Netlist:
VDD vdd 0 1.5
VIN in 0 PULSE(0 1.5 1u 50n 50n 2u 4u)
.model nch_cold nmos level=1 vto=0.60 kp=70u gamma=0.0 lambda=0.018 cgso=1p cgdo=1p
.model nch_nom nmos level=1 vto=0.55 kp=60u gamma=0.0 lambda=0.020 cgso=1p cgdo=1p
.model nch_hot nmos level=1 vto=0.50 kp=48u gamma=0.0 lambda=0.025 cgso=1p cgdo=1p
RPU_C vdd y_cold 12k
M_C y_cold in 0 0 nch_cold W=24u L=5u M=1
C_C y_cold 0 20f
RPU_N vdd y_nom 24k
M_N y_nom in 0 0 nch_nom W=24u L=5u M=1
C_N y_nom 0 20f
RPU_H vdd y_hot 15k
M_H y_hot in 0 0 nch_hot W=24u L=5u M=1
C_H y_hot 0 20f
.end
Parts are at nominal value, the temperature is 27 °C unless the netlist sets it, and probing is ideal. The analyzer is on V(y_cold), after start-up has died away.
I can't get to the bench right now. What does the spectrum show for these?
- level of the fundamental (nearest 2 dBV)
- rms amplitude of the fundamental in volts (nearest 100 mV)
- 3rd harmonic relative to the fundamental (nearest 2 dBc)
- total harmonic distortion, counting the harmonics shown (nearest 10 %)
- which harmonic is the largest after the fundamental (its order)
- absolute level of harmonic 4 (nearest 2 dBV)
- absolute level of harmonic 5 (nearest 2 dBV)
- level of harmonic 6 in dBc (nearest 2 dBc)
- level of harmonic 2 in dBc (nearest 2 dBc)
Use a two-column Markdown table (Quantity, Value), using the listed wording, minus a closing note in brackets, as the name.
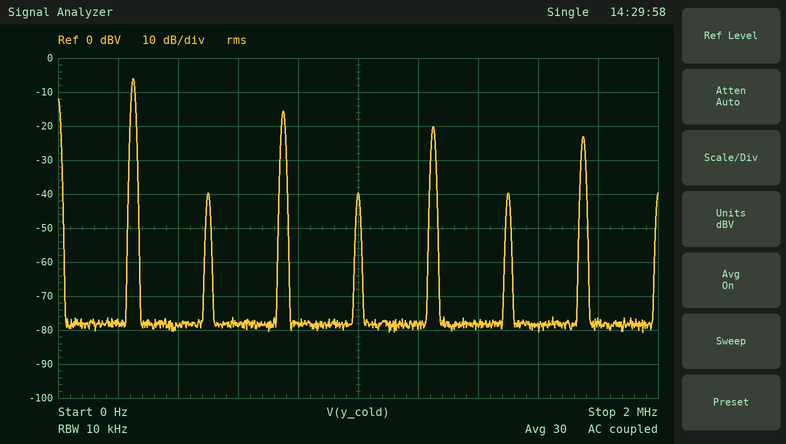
| Quantity | Value |
|---|---|
| level of the fundamental | -6 dBV |
| rms amplitude of the fundamental in volts | 500 mV |
| 3rd harmonic relative to the fundamental | -10 dBc |
| total harmonic distortion, counting the harmonics shown | 40 % |
| which harmonic is the largest after the fundamental | 3 |
| absolute level of harmonic 4 | -40 dBV |
| absolute level of harmonic 5 | -20 dBV |
| level of harmonic 6 in dBc | -34 dBc |
| level of harmonic 2 in dBc | -34 dBc |
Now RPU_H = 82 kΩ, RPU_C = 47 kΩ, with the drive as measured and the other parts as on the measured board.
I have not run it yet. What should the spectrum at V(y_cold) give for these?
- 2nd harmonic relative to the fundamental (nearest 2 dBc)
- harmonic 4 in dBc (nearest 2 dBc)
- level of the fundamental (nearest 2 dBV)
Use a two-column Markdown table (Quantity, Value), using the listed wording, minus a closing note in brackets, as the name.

| Quantity | Value |
|---|---|
| 2nd harmonic relative to the fundamental | -30 dBc |
| harmonic 4 in dBc | -30 dBc |
| level of the fundamental | -4 dBV |
